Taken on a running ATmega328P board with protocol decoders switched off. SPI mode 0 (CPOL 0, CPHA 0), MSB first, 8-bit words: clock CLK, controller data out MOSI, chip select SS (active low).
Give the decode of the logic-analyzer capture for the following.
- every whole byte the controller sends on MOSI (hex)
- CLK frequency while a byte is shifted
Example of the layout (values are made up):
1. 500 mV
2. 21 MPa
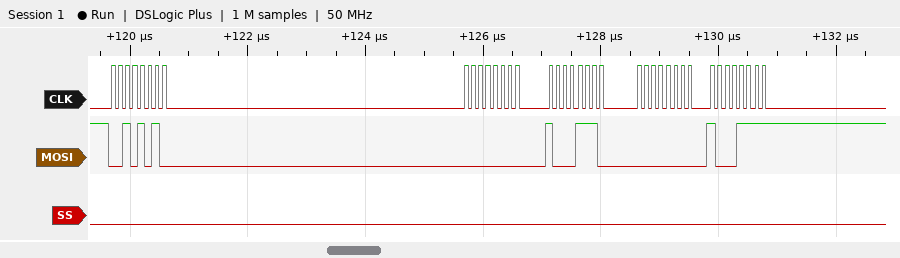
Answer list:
1. 2A 00 8E 00 8F
2. 8 MHz
